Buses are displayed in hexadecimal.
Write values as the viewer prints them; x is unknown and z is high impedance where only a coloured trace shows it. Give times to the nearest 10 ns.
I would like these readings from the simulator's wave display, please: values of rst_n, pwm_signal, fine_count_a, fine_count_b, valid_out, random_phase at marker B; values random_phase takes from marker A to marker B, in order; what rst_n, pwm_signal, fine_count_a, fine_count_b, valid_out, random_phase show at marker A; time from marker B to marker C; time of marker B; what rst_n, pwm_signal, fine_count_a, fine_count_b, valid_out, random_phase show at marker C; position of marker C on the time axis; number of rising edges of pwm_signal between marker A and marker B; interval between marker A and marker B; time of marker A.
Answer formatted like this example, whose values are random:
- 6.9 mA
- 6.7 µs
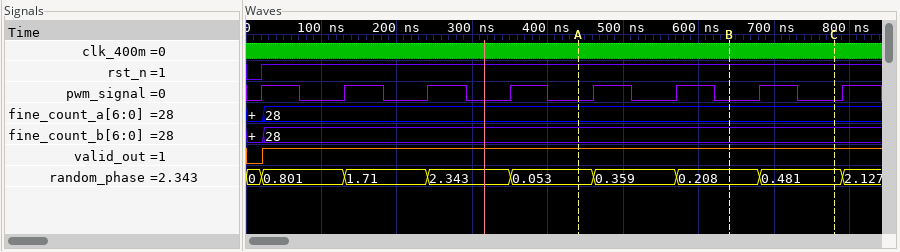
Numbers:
- rst_n=1, pwm_signal=0, fine_count_a=28, fine_count_b=28, valid_out=1, random_phase=0.208
- 0.053, 0.359, 0.208
- rst_n=1, pwm_signal=0, fine_count_a=28, fine_count_b=28, valid_out=1, random_phase=0.053
- 140 ns
- 640 ns
- rst_n=1, pwm_signal=0, fine_count_a=28, fine_count_b=28, valid_out=1, random_phase=0.481
- 780 ns
- 2
- 200 ns
- 440 ns
